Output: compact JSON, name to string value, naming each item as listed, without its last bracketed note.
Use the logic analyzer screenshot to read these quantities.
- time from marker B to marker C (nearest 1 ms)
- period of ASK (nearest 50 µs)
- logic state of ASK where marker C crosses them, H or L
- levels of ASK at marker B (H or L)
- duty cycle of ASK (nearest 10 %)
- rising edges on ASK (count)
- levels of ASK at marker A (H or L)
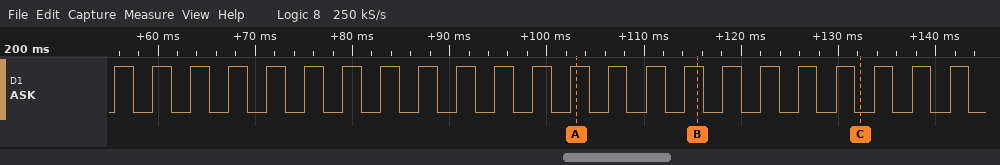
{"time from marker B to marker C": "17 ms", "period of ASK": "3900 µs", "logic state of ASK where marker C crosses them, H or L": "ASK=L", "levels of ASK at marker B": "ASK=H", "duty cycle of ASK": "50 %", "rising edges on ASK": "23", "levels of ASK at marker A": "ASK=H"}
